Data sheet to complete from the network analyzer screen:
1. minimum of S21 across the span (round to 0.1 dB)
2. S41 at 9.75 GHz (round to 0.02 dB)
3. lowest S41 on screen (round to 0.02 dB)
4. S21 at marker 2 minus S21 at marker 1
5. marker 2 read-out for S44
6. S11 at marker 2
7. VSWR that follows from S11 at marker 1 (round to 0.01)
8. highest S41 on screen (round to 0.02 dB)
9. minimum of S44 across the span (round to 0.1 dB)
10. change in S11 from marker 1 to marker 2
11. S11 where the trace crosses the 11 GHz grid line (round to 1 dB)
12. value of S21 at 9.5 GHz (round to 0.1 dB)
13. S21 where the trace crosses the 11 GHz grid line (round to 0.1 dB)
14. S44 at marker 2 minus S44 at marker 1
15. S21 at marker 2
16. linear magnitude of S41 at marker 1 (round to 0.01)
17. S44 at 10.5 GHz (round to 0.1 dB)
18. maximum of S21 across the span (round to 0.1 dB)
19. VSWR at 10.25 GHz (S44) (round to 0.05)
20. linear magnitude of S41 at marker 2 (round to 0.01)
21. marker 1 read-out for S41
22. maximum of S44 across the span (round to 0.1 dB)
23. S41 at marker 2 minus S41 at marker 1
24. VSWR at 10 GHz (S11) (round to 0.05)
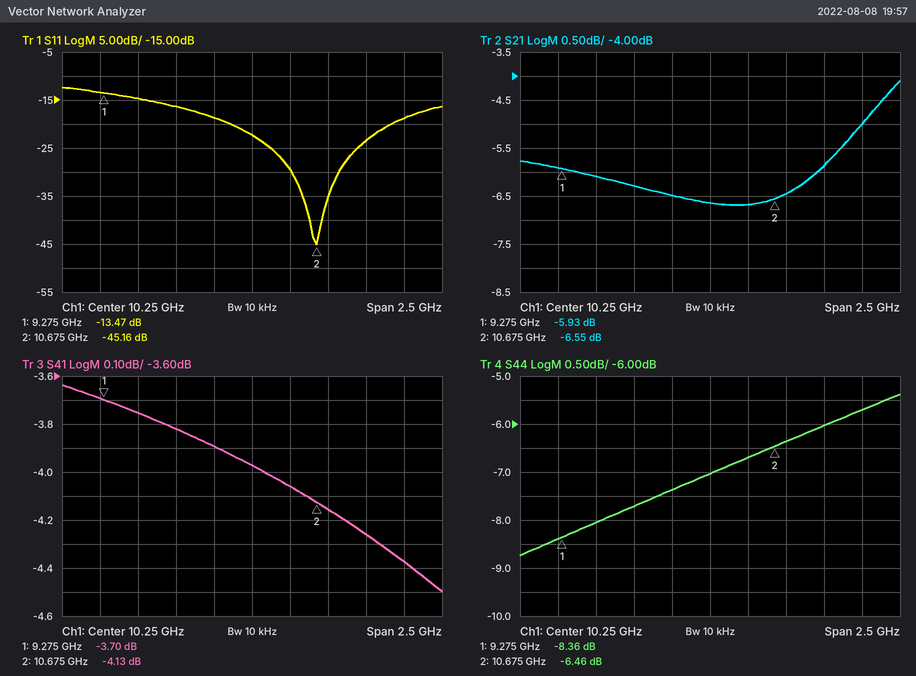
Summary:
-6.7 dB
-3.82 dB
-4.50 dB
-0.62 dB
-6.46 dB
-45.16 dB
1.54
-3.64 dB
-8.7 dB
-31.69 dB
-23 dB
-6.1 dB
-5.9 dB
1.90 dB
-6.55 dB
0.65
-6.7 dB
-4.1 dB
2.60
0.62
-3.70 dB
-5.4 dB
-0.43 dB
1.25
